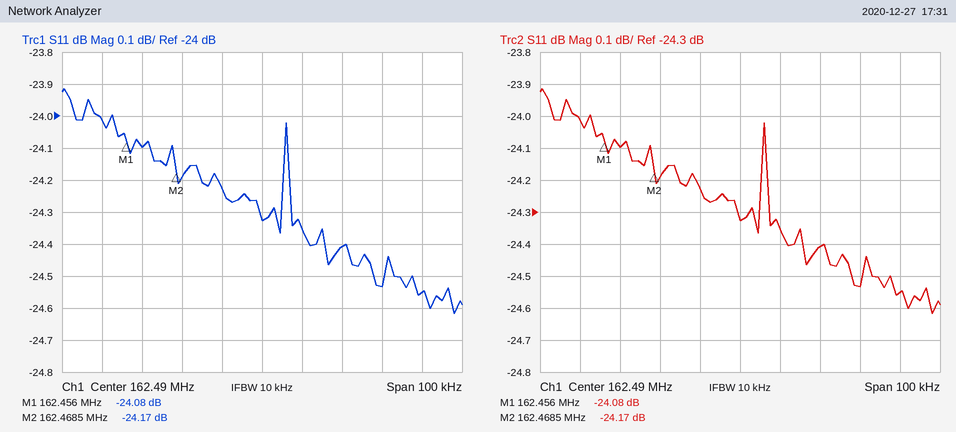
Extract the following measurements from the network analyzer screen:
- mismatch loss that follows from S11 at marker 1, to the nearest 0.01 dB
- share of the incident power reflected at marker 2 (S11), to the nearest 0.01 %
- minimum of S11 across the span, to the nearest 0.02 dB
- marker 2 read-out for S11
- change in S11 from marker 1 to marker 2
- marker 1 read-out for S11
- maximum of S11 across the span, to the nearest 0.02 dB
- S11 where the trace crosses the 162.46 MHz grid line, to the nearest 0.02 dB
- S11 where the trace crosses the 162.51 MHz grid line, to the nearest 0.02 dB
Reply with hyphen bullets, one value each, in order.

- 0.02 dB
- 0.38 %
- -24.62 dB
- -24.17 dB
- -0.09 dB
- -24.08 dB
- -23.92 dB
- -24.10 dB
- -24.40 dB
